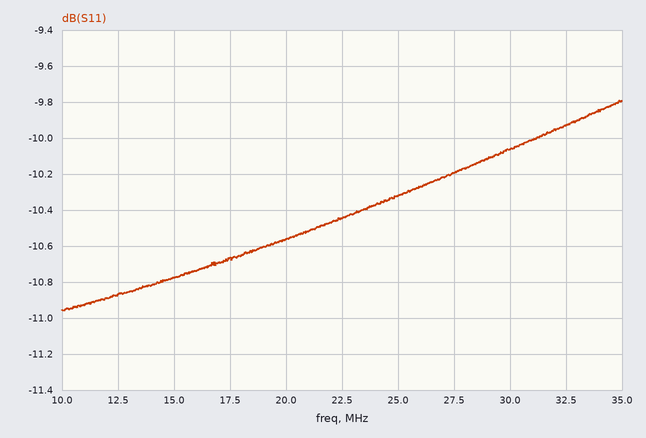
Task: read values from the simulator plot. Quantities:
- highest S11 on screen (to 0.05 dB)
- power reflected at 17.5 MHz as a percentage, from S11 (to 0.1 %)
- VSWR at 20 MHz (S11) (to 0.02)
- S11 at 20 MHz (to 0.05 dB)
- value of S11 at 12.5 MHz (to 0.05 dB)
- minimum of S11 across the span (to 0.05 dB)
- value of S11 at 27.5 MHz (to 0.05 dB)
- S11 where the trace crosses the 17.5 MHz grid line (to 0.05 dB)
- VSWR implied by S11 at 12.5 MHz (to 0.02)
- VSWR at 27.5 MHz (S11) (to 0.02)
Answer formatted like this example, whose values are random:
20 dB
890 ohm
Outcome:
-9.80 dB
8.6 %
1.84
-10.55 dB
-10.85 dB
-10.95 dB
-10.20 dB
-10.65 dB
1.80
1.90
